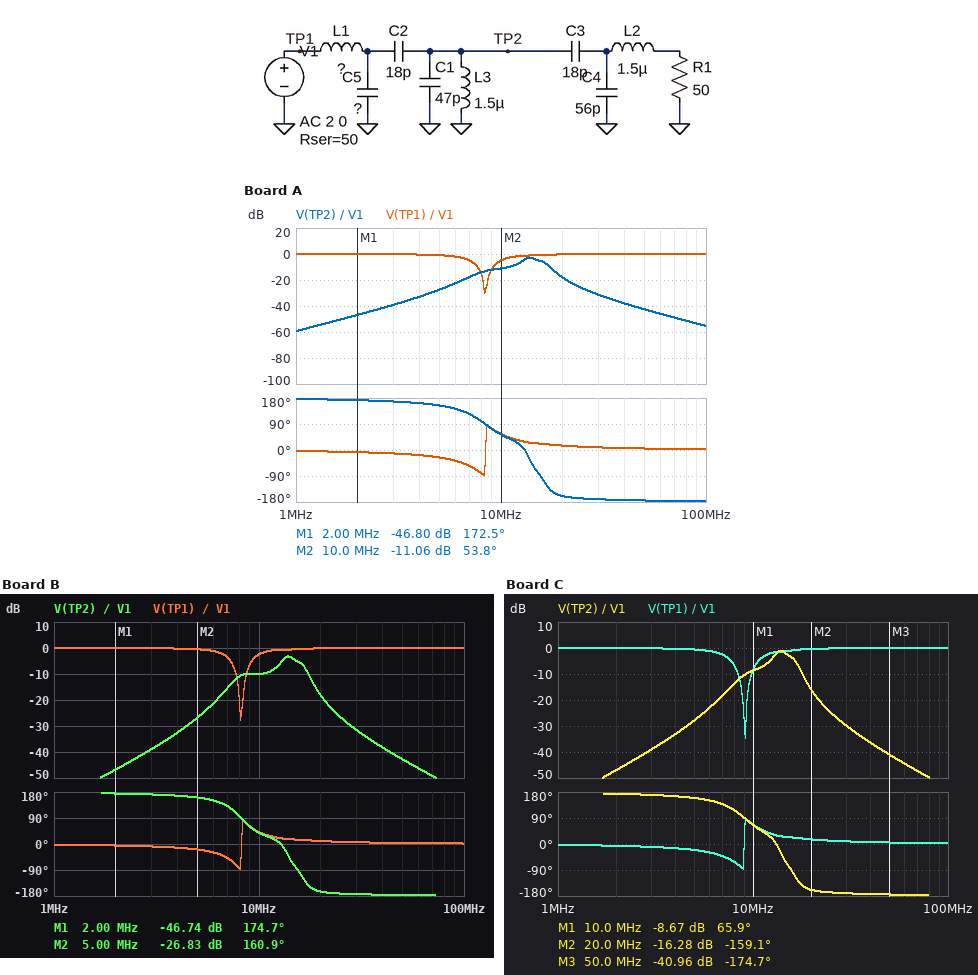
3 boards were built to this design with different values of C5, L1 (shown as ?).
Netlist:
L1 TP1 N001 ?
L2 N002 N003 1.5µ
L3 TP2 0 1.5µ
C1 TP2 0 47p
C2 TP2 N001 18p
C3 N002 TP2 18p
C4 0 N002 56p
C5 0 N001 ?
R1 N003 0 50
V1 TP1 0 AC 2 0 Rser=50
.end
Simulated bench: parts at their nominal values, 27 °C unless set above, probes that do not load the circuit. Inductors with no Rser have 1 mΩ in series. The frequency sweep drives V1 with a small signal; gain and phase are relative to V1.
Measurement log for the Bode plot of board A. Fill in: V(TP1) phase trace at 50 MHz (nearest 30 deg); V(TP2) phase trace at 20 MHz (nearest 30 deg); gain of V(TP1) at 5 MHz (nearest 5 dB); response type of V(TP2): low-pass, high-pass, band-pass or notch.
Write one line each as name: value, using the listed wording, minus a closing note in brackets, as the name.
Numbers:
V(TP1) phase trace at 50 MHz: 0 deg
V(TP2) phase trace at 20 MHz: -150 deg
gain of V(TP1) at 5 MHz: 0 dB
response type of V(TP2): low-pass, high-pass, band-pass or notch: band-pass
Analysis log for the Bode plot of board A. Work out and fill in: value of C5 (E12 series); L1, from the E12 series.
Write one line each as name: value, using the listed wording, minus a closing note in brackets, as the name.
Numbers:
value of C5: 180 pF
L1, from the E12 series: 1.8 µH
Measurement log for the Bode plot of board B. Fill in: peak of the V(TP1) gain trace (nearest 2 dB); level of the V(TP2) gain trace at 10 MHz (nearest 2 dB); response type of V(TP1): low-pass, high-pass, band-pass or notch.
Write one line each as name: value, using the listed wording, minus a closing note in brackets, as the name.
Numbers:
peak of the V(TP1) gain trace: 0 dB
level of the V(TP2) gain trace at 10 MHz: -10 dB
response type of V(TP1): low-pass, high-pass, band-pass or notch: notch
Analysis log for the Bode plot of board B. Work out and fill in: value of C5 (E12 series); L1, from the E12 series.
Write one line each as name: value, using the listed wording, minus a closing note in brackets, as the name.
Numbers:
value of C5: 120 pF
L1, from the E12 series: 2.7 µH
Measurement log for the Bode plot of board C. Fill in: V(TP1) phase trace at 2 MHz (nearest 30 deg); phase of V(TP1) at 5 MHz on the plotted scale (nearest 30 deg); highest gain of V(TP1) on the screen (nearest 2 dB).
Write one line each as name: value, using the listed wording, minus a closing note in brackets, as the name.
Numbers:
V(TP1) phase trace at 2 MHz: 0 deg
phase of V(TP1) at 5 MHz on the plotted scale: -30 deg
highest gain of V(TP1) on the screen: 0 dB
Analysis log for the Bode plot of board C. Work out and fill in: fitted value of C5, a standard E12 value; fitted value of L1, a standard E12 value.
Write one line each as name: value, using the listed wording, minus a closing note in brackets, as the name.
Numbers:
fitted value of C5, a standard E12 value: 150 pF
fitted value of L1, a standard E12 value: 1.8 µH
